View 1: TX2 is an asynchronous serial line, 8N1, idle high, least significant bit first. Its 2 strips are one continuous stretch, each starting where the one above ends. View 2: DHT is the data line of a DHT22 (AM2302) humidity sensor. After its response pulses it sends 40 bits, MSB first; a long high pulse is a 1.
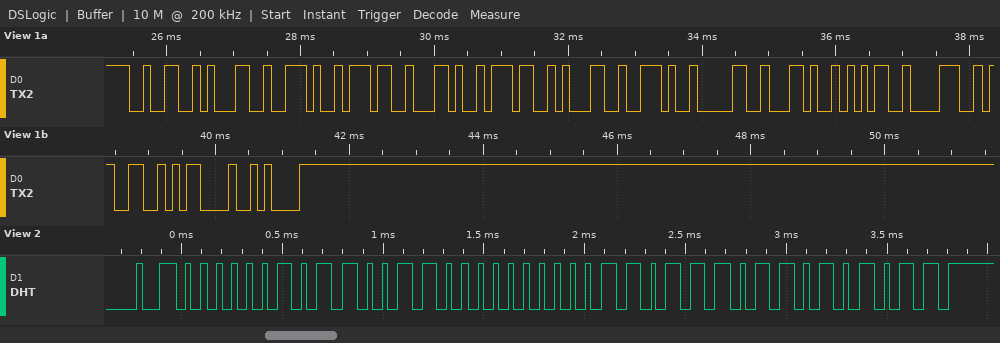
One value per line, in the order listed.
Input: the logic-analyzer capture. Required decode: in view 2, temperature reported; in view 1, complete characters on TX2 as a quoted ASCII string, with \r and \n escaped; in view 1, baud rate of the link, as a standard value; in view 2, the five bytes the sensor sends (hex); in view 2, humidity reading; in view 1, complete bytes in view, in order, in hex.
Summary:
22.1 °C
"21.7,71.0,583\r\n"
9600 baud
02 CC 00 DD AB
71.6 %
32 31 2E 37 2C 37 31 2E 30 2C 35 38 33 0D 0A
